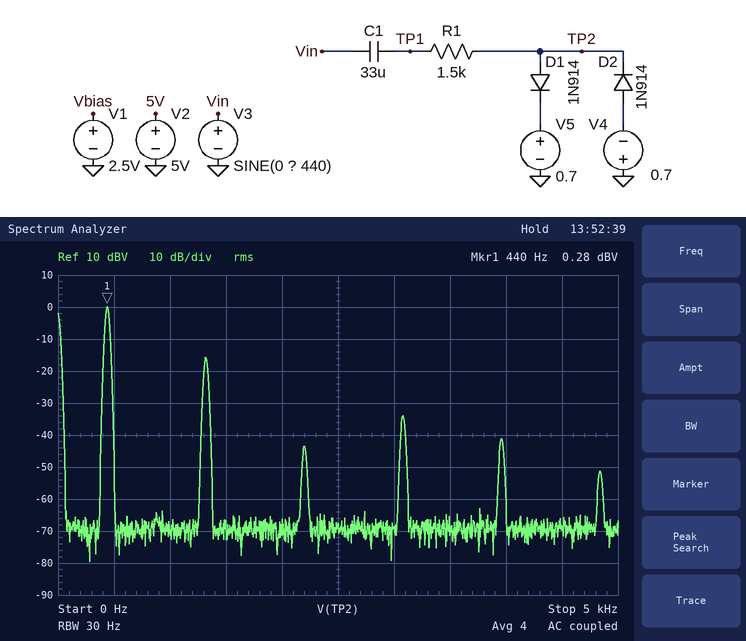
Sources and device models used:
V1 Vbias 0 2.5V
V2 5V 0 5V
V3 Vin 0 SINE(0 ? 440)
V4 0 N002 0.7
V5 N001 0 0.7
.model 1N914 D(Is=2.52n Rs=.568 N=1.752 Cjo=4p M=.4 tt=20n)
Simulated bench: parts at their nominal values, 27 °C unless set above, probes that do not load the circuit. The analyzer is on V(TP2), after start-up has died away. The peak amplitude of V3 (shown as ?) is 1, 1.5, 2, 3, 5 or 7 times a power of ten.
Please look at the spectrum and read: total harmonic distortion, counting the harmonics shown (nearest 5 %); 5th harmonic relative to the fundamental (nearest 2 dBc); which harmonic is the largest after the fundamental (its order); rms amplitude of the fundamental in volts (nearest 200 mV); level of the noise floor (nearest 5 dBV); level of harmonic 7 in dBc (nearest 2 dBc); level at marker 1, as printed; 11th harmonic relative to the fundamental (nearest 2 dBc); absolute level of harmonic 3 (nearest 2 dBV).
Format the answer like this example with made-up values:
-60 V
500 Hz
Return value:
15 %
-44 dBc
3
1.0 V
-70 dBV
-34 dBc
0.28 dBV
-52 dBc
-16 dBV
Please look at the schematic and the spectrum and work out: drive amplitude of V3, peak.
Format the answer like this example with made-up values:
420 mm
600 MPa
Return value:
2 V
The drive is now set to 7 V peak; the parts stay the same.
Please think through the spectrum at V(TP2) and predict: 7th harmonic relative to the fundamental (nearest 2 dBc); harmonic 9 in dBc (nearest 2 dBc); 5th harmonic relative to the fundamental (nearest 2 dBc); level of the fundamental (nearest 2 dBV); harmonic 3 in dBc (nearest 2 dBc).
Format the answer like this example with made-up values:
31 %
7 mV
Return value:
-20 dBc
-24 dBc
-16 dBc
2 dBV
-10 dBc
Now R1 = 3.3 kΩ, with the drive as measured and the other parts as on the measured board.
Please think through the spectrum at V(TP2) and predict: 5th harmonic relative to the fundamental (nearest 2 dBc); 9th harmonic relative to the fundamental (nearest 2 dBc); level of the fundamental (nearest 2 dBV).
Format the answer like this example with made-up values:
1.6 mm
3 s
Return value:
-38 dBc
-40 dBc
0 dBV
